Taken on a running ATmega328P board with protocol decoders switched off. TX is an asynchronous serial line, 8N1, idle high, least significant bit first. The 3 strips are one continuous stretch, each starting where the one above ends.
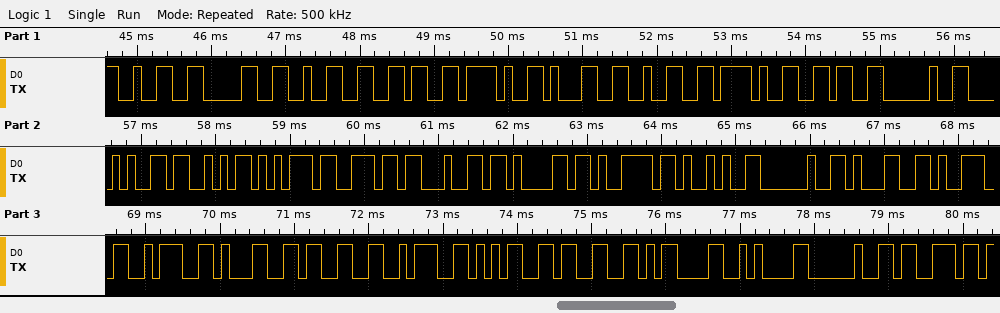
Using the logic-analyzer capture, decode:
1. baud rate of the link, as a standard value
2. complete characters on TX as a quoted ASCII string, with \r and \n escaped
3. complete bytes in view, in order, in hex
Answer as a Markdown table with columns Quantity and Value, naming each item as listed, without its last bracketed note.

| Quantity | Value |
|---|---|
| baud rate of the link, as a standard value | 9600 baud |
| complete characters on TX as a quoted ASCII string, with \r and \n escaped | "2026/12/6 (Sunday) 19:13:53\r\n s" |
| complete bytes in view, in order, in hex | 32 30 32 36 2F 31 32 2F 36 20 28 53 75 6E 64 61 79 29 20 31 39 3A 31 33 3A 35 33 0D 0A 20 73 |
